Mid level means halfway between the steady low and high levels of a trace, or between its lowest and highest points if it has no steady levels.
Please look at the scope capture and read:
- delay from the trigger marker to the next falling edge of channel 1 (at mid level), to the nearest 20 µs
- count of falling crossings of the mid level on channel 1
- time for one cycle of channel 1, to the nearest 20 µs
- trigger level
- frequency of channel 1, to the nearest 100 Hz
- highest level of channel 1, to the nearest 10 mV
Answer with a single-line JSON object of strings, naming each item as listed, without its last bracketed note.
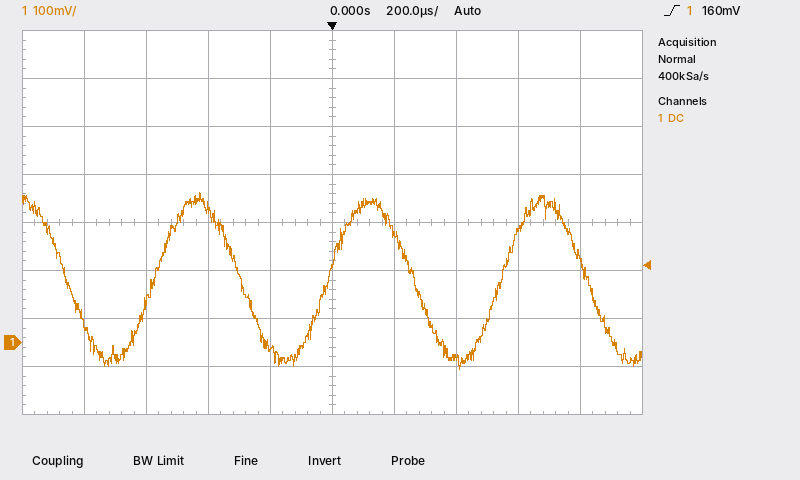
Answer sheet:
{"delay from the trigger marker to the next falling edge of channel 1 (at mid level), to the nearest 20 µs": "260 µs", "count of falling crossings of the mid level on channel 1": "4", "time for one cycle of channel 1, to the nearest 20 µs": "560 µs", "trigger level": "160 mV", "frequency of channel 1, to the nearest 100 Hz": "1.8 kHz", "highest level of channel 1, to the nearest 10 mV": "310 mV"}
